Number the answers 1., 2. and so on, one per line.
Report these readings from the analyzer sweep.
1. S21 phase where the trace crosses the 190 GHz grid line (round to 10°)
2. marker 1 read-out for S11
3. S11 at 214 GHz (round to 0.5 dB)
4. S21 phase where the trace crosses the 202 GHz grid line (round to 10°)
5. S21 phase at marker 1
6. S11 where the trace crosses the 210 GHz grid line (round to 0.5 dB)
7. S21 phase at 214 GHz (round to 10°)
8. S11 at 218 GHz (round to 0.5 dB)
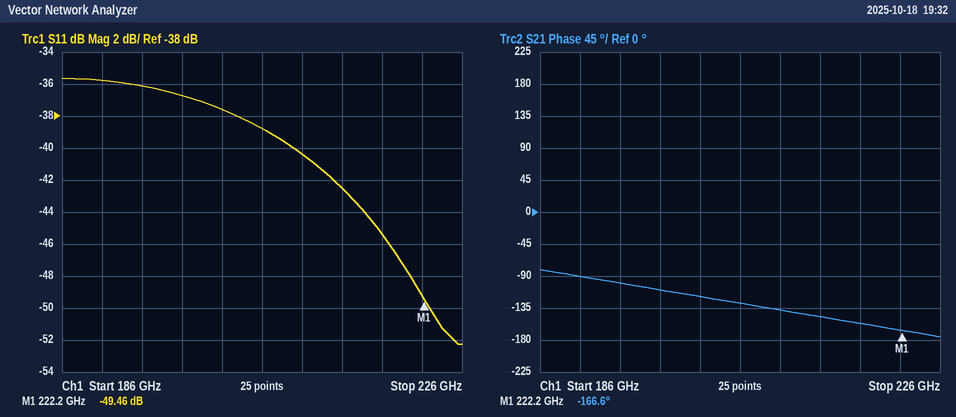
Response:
1. -90°
2. -49.46 dB
3. -42.5 dB
4. -120°
5. -166.6°
6. -40.5 dB
7. -150°
8. -45.5 dB
